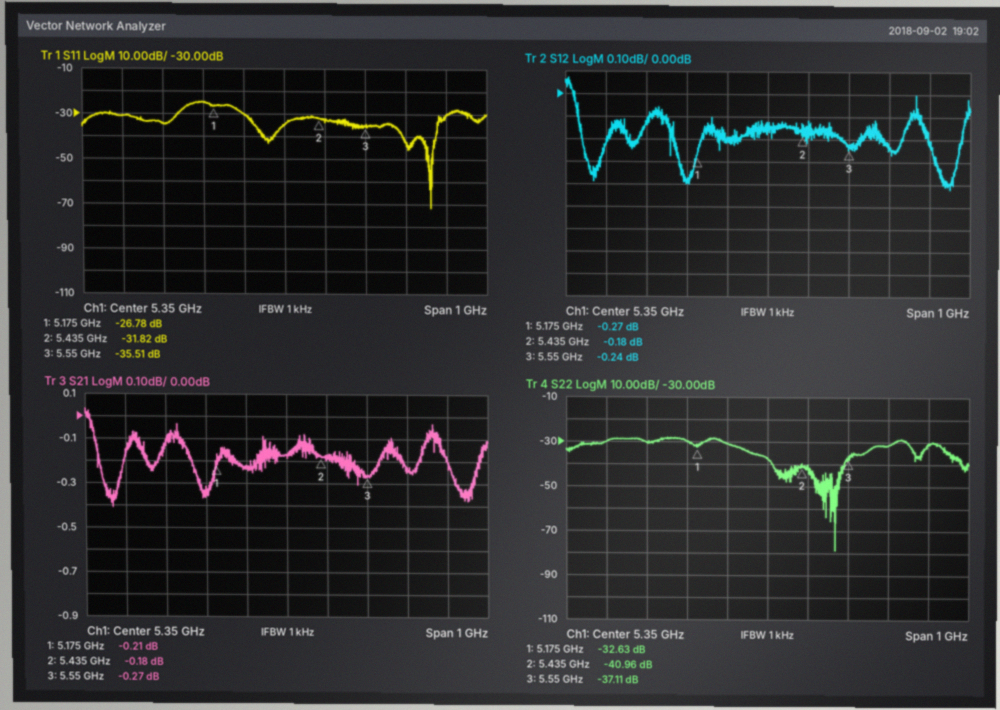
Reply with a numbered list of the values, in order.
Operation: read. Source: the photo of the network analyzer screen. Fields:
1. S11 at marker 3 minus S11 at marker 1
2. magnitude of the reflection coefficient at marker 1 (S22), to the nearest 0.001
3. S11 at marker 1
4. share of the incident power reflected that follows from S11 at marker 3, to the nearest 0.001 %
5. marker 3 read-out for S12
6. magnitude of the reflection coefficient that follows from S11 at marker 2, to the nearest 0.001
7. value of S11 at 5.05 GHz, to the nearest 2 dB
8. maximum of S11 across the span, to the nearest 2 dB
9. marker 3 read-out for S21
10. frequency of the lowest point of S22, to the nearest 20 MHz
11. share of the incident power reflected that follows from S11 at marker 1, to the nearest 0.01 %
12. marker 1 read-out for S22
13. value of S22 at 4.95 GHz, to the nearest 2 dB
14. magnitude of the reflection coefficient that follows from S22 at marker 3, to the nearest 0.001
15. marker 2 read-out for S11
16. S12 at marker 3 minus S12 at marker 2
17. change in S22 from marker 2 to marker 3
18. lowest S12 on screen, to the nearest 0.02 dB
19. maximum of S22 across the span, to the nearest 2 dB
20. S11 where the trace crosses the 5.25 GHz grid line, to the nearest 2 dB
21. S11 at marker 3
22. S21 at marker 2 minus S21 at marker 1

1. -8.73 dB
2. 0.023
3. -26.78 dB
4. 0.028 %
5. -0.24 dB
6. 0.026
7. -34 dB
8. -24 dB
9. -0.27 dB
10. 5.52 GHz
11. 0.21 %
12. -32.63 dB
13. -30 dB
14. 0.014
15. -31.82 dB
16. -0.06 dB
17. 3.85 dB
18. -0.42 dB
19. -28 dB
20. -30 dB
21. -35.51 dB
22. 0.03 dB
